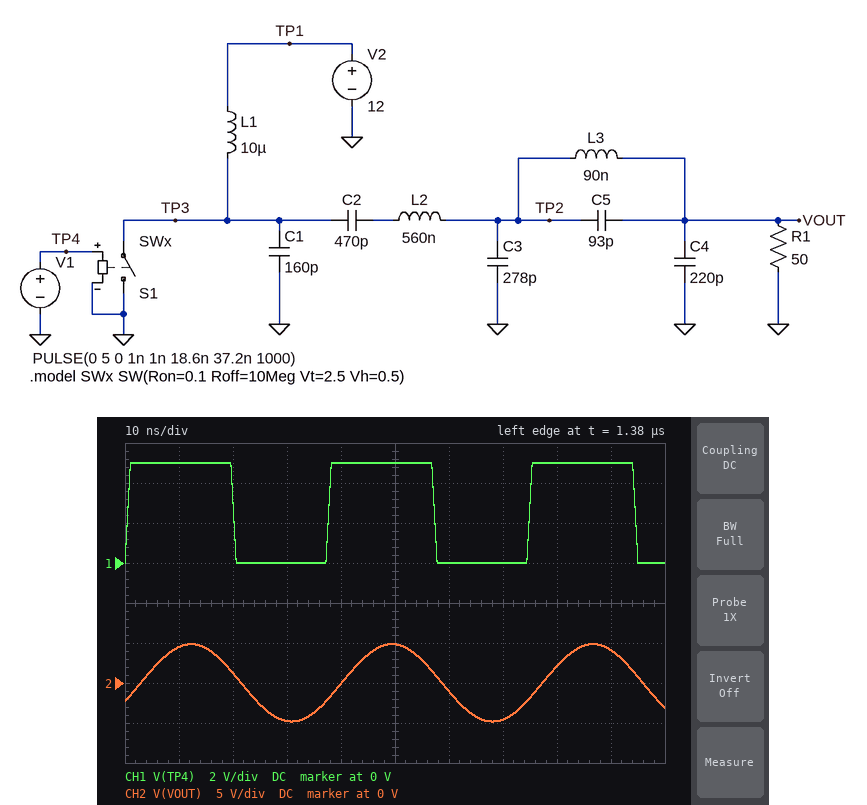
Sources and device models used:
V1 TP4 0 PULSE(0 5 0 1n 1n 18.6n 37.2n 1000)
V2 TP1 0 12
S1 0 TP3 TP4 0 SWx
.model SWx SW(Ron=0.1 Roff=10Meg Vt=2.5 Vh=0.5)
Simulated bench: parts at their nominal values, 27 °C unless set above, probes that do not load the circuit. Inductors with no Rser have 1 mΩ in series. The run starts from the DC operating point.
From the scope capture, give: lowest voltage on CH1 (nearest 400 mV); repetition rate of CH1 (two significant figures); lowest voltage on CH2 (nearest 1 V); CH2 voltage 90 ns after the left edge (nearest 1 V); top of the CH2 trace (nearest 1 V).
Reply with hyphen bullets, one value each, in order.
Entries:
- 0 V
- 27 MHz
- -5 V
- 4 V
- 5 V
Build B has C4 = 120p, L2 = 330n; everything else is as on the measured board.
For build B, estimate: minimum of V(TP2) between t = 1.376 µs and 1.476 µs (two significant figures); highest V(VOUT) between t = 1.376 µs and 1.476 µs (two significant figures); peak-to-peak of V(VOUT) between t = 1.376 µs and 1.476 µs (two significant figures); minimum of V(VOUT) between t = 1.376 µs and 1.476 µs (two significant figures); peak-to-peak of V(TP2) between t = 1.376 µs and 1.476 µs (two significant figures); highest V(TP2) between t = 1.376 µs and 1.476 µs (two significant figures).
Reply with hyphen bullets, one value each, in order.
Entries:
- -8.4 V
- 12 V
- 24 V
- -12 V
- 17 V
- 8.9 V
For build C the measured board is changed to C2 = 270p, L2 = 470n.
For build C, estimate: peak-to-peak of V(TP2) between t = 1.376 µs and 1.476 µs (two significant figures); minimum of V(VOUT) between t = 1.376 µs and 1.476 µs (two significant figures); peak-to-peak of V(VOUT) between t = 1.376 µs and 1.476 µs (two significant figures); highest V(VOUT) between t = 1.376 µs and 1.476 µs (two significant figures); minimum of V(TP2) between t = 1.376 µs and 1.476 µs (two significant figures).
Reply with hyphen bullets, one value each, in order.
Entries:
- 6.9 V
- -7.0 V
- 14 V
- 7.1 V
- -3.0 V
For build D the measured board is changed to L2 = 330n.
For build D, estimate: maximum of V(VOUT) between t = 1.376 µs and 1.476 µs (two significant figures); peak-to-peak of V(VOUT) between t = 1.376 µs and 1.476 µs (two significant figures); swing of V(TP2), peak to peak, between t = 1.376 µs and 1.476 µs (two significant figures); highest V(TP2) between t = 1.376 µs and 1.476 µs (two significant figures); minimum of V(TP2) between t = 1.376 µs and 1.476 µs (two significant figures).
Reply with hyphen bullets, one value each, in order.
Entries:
- 9.6 V
- 19 V
- 9.4 V
- 5.4 V
- -4.0 V
